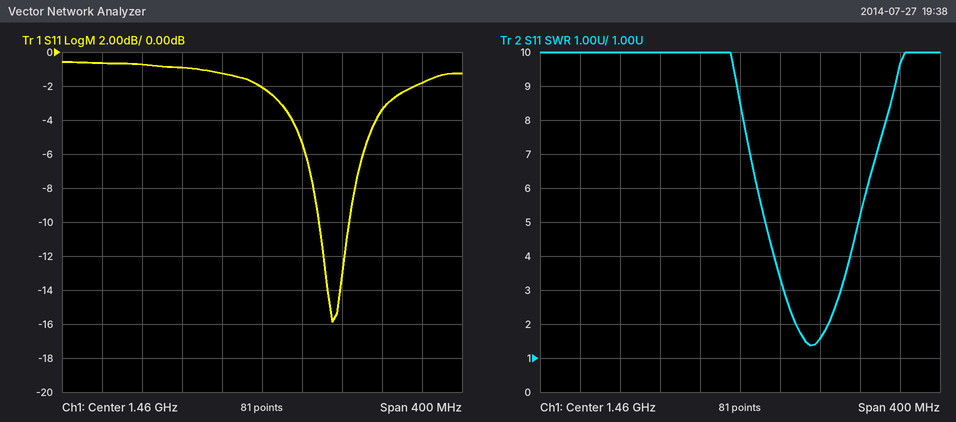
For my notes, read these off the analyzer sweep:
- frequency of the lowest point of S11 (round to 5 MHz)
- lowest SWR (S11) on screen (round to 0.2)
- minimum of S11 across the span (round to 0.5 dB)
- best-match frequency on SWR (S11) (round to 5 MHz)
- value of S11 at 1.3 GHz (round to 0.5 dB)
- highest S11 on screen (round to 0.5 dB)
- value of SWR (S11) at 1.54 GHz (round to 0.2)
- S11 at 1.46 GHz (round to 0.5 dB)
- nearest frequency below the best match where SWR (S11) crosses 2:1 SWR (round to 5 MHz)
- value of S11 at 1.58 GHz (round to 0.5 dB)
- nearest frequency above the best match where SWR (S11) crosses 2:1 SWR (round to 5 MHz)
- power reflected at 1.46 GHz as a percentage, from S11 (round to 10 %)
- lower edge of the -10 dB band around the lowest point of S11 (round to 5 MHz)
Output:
1.530 GHz
1.4
-16.0 dB
1.530 GHz
-0.5 dB
-0.5 dB
1.6
-2.0 dB
1.515 GHz
-3.5 dB
1.550 GHz
60 %
1.515 GHz
